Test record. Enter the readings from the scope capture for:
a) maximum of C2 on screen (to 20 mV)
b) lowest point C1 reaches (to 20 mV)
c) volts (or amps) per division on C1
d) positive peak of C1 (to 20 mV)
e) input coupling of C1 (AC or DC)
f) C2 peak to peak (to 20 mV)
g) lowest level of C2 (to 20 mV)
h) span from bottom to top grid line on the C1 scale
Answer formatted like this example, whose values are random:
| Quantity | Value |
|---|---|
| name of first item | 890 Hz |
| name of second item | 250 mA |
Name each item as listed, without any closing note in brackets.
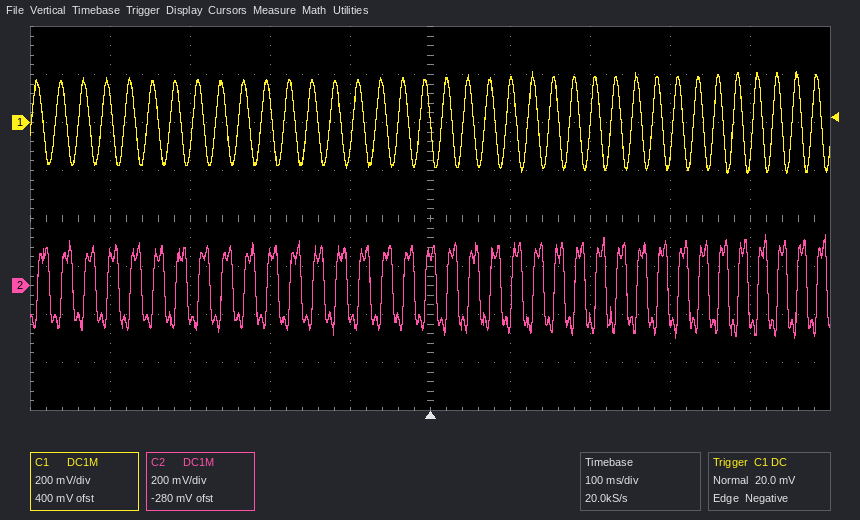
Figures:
| Quantity | Value |
|---|---|
| maximum of C2 on screen | 220 mV |
| lowest point C1 reaches | -220 mV |
| volts (or amps) per division on C1 | 200 mV |
| positive peak of C1 | 220 mV |
| input coupling of C1 | DC |
| C2 peak to peak | 440 mV |
| lowest level of C2 | -220 mV |
| span from bottom to top grid line on the C1 scale | 1.6 V |
